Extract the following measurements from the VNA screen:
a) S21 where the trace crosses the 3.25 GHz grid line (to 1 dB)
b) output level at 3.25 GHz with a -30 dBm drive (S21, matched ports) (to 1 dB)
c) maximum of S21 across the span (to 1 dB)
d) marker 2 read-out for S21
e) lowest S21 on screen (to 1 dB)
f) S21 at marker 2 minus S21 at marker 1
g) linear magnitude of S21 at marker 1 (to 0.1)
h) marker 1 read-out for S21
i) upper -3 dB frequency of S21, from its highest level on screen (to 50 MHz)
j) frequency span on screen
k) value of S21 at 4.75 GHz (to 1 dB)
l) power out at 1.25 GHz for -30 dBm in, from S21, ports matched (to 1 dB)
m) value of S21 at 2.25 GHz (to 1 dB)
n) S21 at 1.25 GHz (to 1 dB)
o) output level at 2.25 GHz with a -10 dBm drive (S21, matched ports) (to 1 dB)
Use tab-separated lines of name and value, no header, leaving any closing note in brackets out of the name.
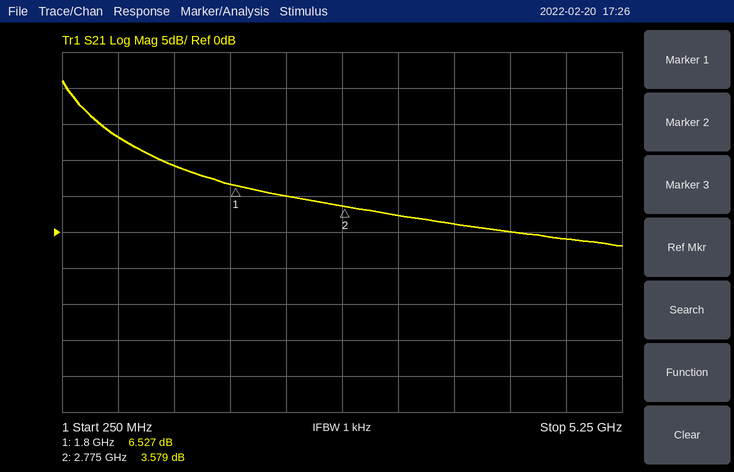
S21 where the trace crosses the 3.25 GHz grid line	2 dB
output level at 3.25 GHz with a -30 dBm drive (S21, matched ports)	-28 dBm
maximum of S21 across the span	21 dB
marker 2 read-out for S21	3.579 dB
lowest S21 on screen	-2 dB
S21 at marker 2 minus S21 at marker 1	-2.948 dB
linear magnitude of S21 at marker 1	2.1
marker 1 read-out for S21	6.527 dB
upper -3 dB frequency of S21, from its highest level on screen	400 MHz
frequency span on screen	5 GHz
value of S21 at 4.75 GHz	-1 dB
power out at 1.25 GHz for -30 dBm in, from S21, ports matched	-21 dBm
value of S21 at 2.25 GHz	5 dB
S21 at 1.25 GHz	9 dB
output level at 2.25 GHz with a -10 dBm drive (S21, matched ports)	-5 dBm
